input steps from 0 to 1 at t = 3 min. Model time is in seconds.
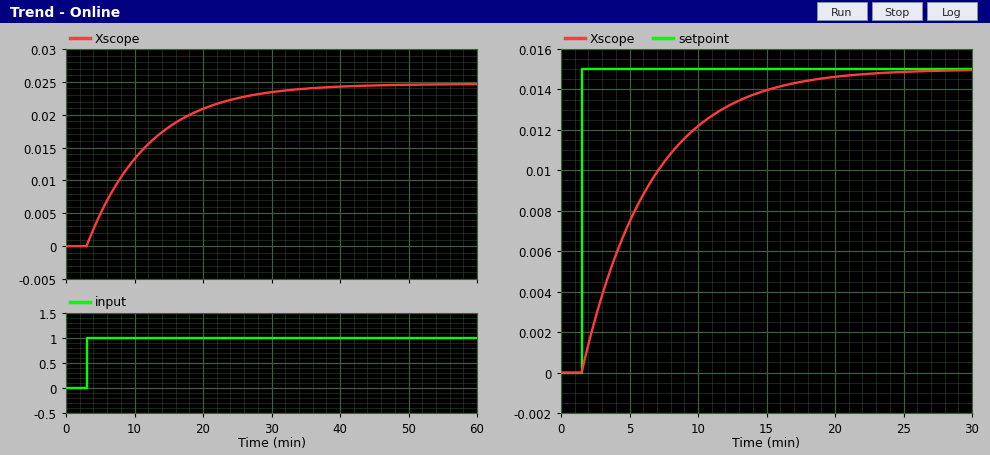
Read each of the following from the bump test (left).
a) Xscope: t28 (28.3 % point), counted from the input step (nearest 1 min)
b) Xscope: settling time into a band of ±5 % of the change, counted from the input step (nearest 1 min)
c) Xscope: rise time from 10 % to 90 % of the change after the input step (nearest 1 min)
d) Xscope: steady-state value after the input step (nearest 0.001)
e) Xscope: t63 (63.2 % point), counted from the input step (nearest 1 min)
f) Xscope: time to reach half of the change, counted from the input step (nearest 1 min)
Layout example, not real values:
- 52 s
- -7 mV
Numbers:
- 3 min
- 27 min
- 20 min
- 0.025
- 9 min
- 6 min
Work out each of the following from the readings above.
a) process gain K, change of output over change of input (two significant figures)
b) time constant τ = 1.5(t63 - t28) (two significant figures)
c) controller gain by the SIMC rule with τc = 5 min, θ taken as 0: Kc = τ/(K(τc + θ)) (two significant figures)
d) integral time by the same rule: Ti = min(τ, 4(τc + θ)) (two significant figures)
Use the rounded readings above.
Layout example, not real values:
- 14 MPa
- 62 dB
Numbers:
- 0.025
- 9.0 min
- 72
- 9.0 min
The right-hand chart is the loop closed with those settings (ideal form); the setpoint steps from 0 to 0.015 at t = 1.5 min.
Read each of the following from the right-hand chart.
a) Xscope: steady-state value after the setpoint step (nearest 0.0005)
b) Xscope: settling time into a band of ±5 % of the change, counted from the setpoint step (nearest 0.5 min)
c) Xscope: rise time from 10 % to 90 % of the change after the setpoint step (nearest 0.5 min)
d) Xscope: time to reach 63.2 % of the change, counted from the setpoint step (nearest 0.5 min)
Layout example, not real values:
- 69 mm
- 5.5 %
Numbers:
- 0.0150
- 15.0 min
- 11.0 min
- 5.0 min
